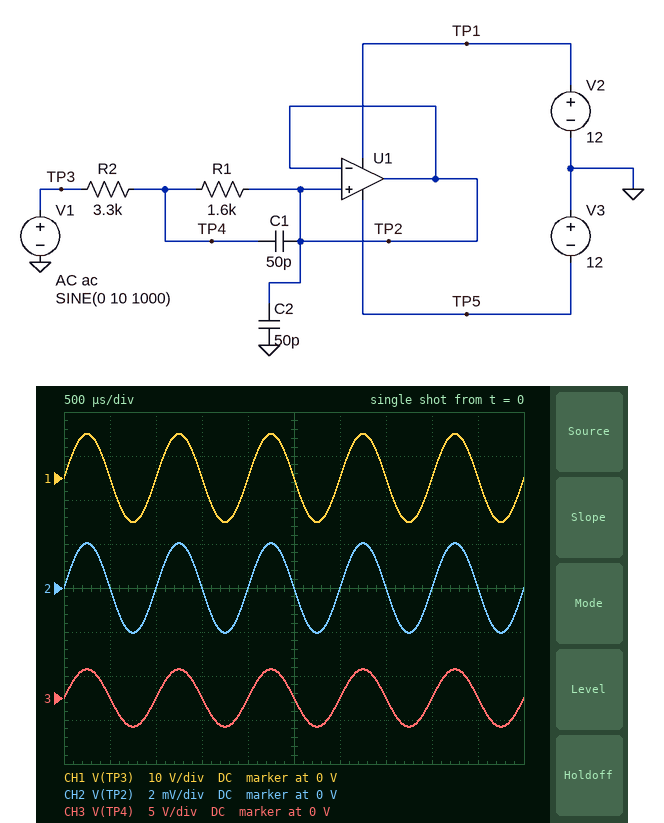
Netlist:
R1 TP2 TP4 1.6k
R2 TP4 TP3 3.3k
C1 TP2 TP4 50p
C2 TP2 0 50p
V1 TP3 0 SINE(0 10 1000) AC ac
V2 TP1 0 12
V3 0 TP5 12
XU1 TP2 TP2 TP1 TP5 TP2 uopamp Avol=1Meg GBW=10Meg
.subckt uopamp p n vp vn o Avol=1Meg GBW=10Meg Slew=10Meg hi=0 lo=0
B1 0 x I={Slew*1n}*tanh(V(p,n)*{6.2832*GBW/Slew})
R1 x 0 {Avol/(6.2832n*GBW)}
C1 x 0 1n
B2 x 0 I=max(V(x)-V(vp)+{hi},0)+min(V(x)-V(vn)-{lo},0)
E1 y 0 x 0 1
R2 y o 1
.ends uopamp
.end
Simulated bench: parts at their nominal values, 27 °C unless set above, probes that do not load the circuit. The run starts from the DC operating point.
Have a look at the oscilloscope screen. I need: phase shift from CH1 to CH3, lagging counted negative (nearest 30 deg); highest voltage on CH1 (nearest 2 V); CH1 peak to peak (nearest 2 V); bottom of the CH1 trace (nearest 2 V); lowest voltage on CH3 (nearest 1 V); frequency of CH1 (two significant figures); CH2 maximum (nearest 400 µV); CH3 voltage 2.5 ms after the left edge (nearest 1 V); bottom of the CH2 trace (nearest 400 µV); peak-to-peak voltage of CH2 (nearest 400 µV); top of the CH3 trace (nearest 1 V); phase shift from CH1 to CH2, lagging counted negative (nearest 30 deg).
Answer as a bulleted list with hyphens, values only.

- 0 deg
- 10 V
- 20 V
- -10 V
- -3 V
- 1.0 kHz
- 2.0 mV
- 0 V
- -2.0 mV
- 4.0 mV
- 3 V
- 0 deg
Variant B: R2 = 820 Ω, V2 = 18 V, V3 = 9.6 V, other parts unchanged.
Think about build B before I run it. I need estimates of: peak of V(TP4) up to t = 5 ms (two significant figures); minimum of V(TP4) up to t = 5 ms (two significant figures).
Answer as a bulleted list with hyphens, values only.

- 6.6 V
- -6.6 V
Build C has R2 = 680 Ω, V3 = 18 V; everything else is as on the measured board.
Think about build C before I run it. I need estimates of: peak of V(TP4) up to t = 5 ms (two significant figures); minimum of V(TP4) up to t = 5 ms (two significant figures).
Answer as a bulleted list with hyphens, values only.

- 7.0 V
- -7.0 V
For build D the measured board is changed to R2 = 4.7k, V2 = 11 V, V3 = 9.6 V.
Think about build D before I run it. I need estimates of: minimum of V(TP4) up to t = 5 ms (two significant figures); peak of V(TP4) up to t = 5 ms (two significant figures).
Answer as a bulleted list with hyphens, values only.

- -2.5 V
- 2.5 V
